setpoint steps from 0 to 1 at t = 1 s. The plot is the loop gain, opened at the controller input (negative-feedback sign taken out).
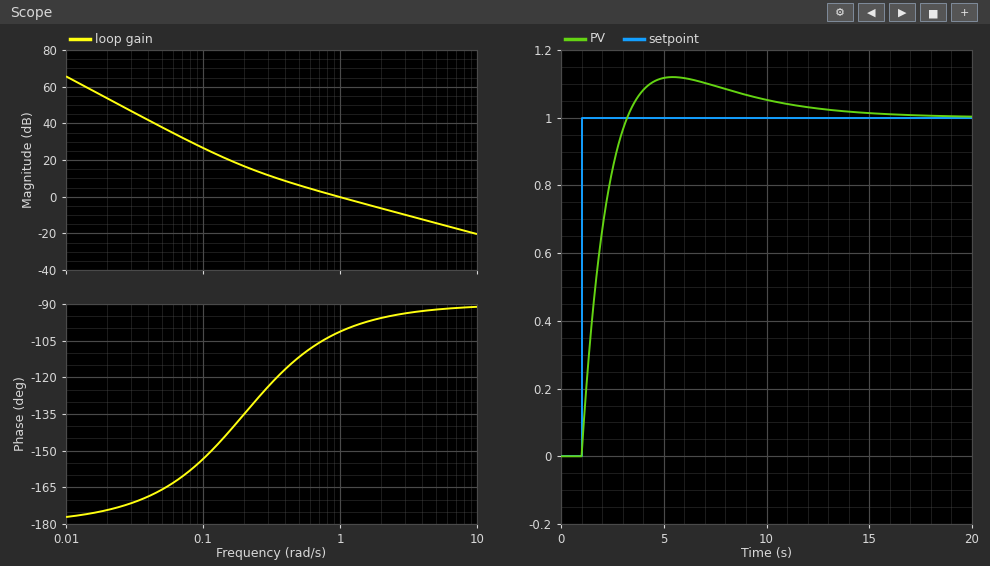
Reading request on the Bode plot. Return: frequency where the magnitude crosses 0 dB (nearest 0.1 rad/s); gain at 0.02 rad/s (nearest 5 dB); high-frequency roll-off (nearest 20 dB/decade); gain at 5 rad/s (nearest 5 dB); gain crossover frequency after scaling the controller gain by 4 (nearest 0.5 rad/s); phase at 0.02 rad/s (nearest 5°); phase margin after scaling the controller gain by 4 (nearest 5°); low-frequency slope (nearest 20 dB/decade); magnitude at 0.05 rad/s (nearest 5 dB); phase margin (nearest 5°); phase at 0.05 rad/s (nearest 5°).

1.0 rad/s
55 dB
-20 dB/decade
-15 dB
4.0 rad/s
-175°
85°
-40 dB/decade
40 dB
80°
-165°
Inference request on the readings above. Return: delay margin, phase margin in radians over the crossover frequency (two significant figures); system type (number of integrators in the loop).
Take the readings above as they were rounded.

1.4 s
2
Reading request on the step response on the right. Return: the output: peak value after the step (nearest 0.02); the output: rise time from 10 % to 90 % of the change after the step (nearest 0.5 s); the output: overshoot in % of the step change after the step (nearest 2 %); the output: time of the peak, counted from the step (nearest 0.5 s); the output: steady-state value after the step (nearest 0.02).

1.12
1.5 s
12 %
4.5 s
1.00
